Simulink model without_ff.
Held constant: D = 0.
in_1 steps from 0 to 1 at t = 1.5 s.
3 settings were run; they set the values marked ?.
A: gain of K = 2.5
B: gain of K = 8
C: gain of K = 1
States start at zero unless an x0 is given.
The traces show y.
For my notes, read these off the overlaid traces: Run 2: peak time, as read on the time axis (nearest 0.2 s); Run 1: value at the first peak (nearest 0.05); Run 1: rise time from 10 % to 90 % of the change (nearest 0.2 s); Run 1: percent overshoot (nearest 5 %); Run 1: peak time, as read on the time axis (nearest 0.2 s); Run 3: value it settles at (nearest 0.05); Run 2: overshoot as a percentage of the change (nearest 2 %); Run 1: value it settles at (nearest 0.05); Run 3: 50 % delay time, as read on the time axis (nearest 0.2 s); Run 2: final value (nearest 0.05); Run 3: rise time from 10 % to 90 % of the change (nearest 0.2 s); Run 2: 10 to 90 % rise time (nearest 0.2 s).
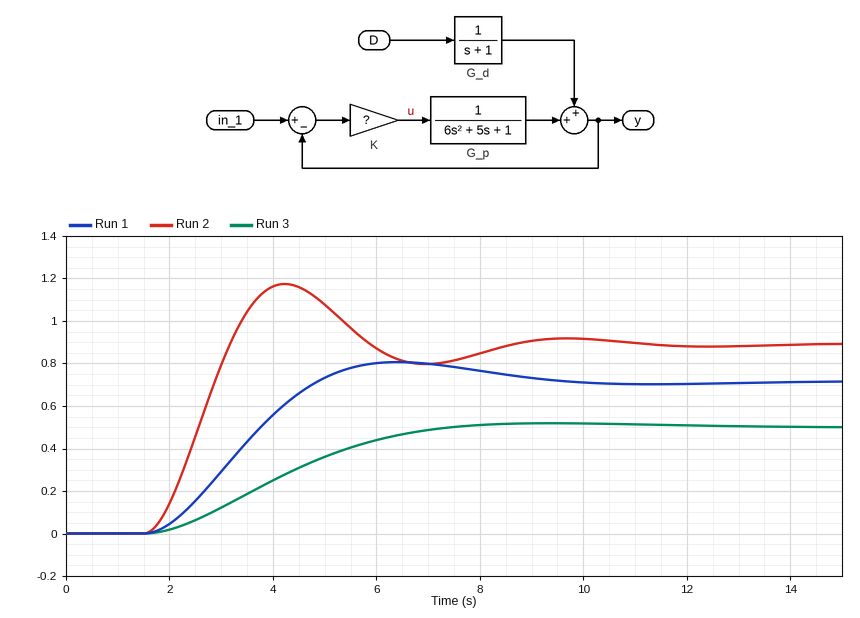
4.2 s
0.80
2.2 s
15 %
6.4 s
0.50
32 %
0.70
4.0 s
0.90
3.8 s
1.2 s
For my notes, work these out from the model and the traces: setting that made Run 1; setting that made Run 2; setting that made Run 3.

A
B
C
